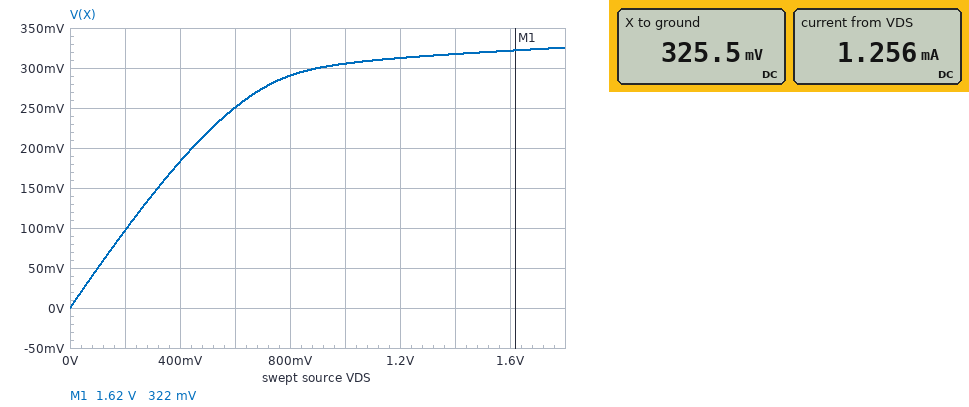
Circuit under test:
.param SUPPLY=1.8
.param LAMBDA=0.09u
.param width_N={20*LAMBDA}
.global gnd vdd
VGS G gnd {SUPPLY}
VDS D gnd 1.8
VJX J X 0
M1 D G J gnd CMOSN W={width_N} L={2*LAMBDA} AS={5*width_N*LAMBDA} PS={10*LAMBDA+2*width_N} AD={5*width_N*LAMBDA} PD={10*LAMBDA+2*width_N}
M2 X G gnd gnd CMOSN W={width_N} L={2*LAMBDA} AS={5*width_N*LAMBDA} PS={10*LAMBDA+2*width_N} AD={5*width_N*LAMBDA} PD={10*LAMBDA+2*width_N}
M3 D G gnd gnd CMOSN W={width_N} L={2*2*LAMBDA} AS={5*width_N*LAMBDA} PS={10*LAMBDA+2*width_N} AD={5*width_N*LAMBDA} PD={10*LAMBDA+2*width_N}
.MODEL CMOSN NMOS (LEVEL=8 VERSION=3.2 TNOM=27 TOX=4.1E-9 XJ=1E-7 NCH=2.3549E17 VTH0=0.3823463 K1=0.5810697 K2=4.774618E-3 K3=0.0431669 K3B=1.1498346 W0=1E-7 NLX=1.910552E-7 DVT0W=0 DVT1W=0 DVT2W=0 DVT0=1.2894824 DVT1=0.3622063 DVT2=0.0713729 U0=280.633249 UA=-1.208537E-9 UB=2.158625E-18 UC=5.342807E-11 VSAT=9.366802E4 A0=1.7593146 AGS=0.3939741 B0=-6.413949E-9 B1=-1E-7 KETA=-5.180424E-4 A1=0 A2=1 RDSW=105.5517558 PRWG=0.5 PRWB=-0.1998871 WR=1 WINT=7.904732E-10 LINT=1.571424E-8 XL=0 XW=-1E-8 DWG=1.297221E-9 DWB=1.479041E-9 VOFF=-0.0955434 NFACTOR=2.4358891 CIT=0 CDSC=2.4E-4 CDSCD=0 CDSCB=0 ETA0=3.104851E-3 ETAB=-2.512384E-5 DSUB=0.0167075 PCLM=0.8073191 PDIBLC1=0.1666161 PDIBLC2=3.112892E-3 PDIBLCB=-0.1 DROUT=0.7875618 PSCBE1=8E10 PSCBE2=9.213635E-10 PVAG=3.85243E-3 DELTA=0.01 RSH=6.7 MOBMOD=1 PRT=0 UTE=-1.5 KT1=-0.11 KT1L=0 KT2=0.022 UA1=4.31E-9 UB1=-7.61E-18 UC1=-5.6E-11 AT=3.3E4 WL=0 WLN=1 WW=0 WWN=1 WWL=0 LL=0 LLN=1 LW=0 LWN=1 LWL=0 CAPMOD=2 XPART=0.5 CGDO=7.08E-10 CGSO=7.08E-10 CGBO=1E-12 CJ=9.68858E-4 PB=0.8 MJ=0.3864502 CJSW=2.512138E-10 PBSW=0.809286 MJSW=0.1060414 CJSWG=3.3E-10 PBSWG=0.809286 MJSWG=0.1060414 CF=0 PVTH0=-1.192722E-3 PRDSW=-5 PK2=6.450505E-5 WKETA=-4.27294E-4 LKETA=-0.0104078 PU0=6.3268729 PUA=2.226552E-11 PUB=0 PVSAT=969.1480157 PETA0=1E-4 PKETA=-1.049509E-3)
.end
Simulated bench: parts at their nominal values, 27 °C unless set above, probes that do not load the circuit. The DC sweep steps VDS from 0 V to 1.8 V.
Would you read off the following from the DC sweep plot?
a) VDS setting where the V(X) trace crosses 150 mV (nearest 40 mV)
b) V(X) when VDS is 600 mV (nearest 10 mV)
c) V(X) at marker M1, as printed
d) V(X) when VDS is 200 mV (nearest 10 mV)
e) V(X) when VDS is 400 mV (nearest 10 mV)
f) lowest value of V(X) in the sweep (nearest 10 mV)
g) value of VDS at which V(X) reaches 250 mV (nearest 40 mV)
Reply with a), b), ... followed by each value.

a) 320 mV
b) 250 mV
c) 322 mV
d) 100 mV
e) 180 mV
f) 0 V
g) 600 mV
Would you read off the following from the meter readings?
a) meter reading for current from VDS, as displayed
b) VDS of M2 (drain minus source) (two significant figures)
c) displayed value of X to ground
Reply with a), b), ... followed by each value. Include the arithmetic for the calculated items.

a) 1.256 mA
b) 325.5 mV = 330 mV
c) 325.5 mV
